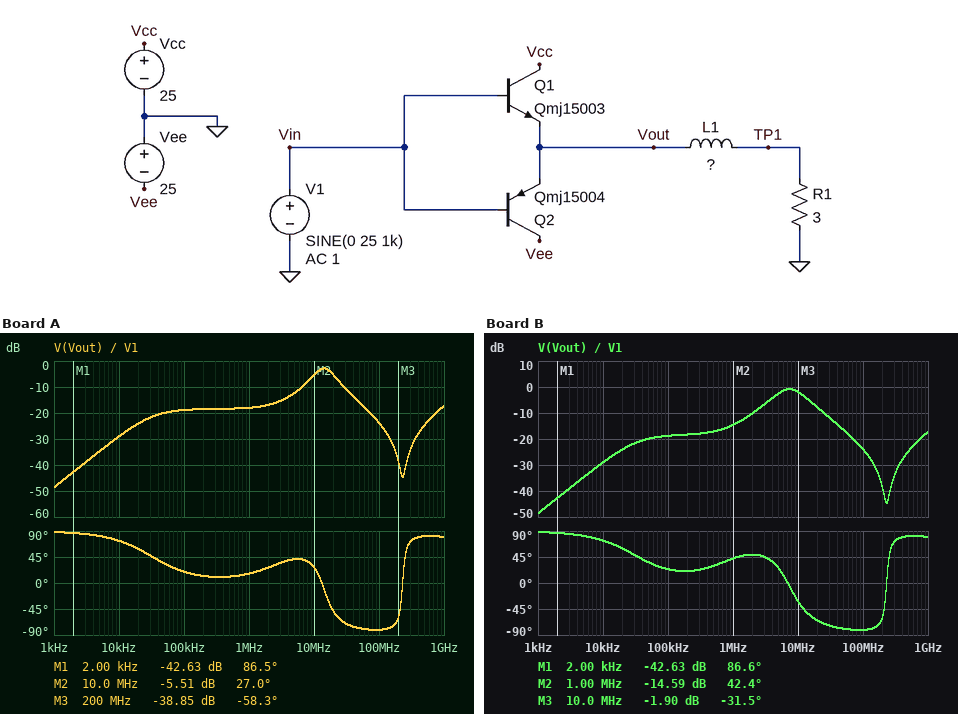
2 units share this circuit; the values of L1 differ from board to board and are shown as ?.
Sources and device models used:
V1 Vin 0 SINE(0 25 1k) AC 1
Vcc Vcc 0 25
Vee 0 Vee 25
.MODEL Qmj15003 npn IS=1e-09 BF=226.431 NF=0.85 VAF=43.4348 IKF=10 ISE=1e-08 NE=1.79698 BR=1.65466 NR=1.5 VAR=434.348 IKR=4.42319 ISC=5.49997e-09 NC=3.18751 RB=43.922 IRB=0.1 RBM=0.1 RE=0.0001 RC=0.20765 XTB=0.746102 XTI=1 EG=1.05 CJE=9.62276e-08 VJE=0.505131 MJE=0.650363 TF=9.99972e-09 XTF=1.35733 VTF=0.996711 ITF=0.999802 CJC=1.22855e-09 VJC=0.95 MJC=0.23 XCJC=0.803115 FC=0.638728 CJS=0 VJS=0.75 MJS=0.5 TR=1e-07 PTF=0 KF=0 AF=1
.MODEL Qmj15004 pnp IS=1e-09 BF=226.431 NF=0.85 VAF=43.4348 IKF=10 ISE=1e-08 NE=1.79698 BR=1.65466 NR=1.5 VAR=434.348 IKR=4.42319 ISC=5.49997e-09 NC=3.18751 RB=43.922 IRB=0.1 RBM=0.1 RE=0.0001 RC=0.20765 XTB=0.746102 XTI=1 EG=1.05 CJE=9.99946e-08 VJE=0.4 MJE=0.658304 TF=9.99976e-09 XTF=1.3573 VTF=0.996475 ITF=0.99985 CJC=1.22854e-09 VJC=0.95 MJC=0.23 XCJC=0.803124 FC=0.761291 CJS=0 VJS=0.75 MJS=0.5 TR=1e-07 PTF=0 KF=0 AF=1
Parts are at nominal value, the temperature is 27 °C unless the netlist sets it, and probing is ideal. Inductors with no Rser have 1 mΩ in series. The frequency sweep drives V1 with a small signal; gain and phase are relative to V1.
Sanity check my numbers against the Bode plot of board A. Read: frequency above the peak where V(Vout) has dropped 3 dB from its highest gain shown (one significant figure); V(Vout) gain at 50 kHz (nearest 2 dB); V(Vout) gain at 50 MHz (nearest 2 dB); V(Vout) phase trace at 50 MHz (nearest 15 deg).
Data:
20 MHz
-20 dB
-16 dB
-75 deg
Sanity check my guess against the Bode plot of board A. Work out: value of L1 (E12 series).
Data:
150 nH
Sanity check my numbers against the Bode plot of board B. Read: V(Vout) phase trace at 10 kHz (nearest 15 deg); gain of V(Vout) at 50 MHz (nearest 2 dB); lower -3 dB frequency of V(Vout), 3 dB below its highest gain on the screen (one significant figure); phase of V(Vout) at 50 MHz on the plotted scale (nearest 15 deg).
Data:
75 deg
-16 dB
4 MHz
-75 deg
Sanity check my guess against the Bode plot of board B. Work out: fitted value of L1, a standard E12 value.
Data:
560 nH
